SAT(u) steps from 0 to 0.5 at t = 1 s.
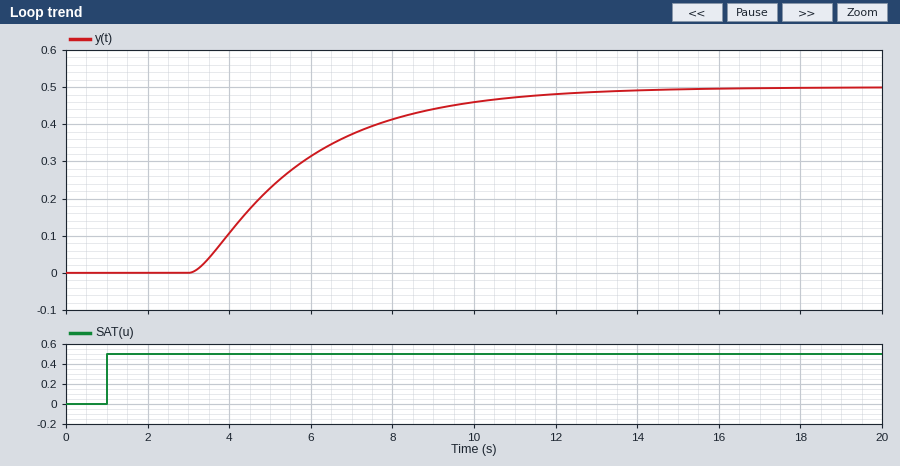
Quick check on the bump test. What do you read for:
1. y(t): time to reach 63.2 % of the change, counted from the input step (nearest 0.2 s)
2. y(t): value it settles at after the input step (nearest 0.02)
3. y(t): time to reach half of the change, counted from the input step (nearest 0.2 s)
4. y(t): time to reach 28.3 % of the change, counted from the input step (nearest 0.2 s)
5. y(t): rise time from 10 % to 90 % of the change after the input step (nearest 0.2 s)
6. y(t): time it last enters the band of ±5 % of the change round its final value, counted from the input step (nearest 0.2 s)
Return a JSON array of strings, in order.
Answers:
["5.0 s", "0.50", "4.2 s", "3.2 s", "5.8 s", "10.2 s"]
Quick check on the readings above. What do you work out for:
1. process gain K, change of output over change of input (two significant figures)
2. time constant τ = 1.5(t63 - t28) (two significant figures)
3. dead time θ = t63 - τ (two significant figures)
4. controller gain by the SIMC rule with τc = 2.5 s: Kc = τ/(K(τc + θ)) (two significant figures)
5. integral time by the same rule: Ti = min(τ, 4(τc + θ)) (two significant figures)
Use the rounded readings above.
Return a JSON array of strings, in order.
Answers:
["1.0", "2.7 s", "2.3 s", "0.56", "2.7 s"]
